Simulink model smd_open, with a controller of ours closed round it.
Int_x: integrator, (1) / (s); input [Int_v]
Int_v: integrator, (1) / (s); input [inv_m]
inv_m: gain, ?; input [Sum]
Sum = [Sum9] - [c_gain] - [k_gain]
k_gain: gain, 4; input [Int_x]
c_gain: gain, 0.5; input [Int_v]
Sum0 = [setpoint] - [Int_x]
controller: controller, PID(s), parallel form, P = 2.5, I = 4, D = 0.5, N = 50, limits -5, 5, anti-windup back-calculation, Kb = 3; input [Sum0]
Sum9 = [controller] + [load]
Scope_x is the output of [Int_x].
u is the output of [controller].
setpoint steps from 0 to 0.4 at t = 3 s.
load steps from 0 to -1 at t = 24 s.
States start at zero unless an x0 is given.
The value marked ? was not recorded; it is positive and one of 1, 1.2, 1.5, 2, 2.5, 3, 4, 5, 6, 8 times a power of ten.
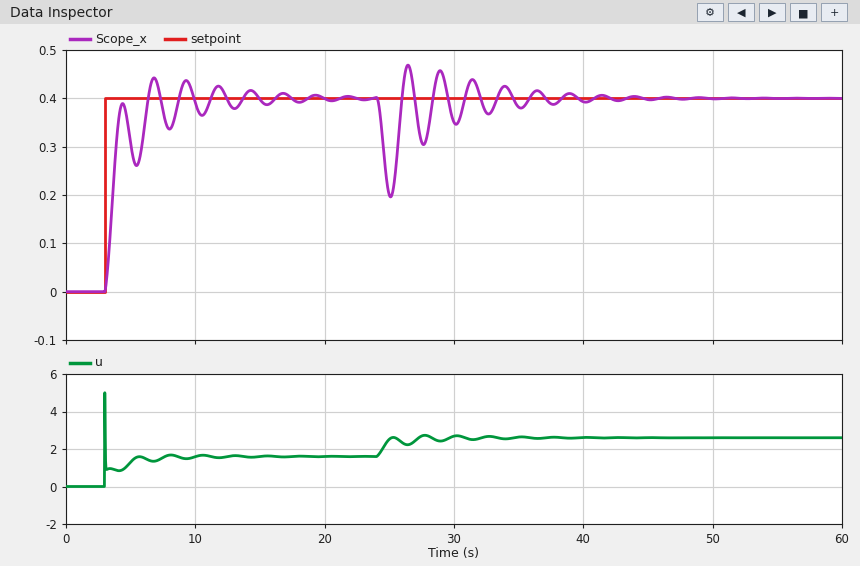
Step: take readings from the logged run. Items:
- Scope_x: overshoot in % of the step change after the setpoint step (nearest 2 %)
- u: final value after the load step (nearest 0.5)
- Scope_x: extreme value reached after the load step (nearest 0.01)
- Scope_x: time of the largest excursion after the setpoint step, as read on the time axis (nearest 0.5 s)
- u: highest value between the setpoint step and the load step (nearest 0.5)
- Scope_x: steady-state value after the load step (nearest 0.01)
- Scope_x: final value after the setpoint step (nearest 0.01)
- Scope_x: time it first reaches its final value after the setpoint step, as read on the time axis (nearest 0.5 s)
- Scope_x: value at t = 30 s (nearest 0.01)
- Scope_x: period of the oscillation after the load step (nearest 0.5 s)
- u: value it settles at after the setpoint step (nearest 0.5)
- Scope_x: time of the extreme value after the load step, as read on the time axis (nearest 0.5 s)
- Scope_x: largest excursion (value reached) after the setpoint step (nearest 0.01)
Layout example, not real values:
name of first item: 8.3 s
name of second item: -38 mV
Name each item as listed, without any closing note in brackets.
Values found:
Scope_x: overshoot in % of the step change after the setpoint step: 10 %
u: final value after the load step: 2.5
Scope_x: extreme value reached after the load step: 0.20
Scope_x: time of the largest excursion after the setpoint step, as read on the time axis: 7.0 s
u: highest value between the setpoint step and the load step: 5.0
Scope_x: steady-state value after the load step: 0.40
Scope_x: final value after the setpoint step: 0.40
Scope_x: time it first reaches its final value after the setpoint step, as read on the time axis: 6.5 s
Scope_x: value at t = 30 s: 0.35
Scope_x: period of the oscillation after the load step: 2.5 s
u: value it settles at after the setpoint step: 1.5
Scope_x: time of the extreme value after the load step, as read on the time axis: 25.0 s
Scope_x: largest excursion (value reached) after the setpoint step: 0.44
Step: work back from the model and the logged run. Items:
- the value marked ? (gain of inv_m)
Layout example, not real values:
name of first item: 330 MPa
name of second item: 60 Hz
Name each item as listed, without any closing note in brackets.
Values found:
the value marked ?: 1
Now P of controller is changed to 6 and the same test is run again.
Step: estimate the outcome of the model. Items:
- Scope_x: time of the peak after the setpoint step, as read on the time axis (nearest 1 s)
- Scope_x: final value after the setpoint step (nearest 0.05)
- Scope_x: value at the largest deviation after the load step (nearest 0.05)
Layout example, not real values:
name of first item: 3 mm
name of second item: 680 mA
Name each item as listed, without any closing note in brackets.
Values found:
Scope_x: time of the peak after the setpoint step, as read on the time axis: 4 s
Scope_x: final value after the setpoint step: 0.40
Scope_x: value at the largest deviation after the load step: 0.25
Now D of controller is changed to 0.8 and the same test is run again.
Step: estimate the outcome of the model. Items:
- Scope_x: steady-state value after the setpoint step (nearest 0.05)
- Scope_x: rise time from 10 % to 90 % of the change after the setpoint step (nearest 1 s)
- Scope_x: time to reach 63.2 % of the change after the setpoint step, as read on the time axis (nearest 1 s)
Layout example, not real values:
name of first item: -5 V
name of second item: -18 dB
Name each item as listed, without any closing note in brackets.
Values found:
Scope_x: steady-state value after the setpoint step: 0.40
Scope_x: rise time from 10 % to 90 % of the change after the setpoint step: 3 s
Scope_x: time to reach 63.2 % of the change after the setpoint step, as read on the time axis: 4 s
